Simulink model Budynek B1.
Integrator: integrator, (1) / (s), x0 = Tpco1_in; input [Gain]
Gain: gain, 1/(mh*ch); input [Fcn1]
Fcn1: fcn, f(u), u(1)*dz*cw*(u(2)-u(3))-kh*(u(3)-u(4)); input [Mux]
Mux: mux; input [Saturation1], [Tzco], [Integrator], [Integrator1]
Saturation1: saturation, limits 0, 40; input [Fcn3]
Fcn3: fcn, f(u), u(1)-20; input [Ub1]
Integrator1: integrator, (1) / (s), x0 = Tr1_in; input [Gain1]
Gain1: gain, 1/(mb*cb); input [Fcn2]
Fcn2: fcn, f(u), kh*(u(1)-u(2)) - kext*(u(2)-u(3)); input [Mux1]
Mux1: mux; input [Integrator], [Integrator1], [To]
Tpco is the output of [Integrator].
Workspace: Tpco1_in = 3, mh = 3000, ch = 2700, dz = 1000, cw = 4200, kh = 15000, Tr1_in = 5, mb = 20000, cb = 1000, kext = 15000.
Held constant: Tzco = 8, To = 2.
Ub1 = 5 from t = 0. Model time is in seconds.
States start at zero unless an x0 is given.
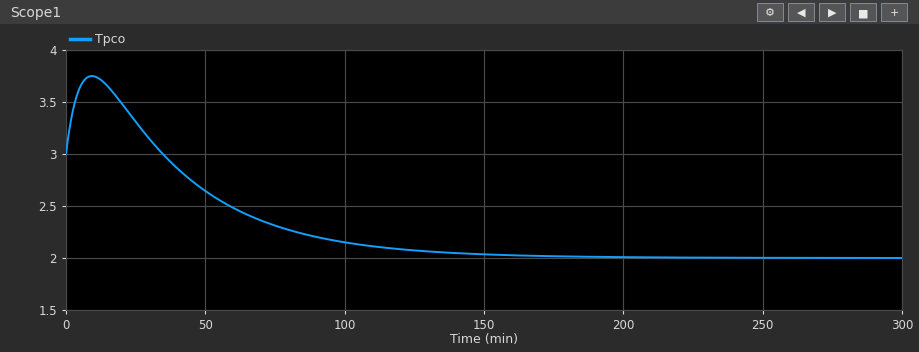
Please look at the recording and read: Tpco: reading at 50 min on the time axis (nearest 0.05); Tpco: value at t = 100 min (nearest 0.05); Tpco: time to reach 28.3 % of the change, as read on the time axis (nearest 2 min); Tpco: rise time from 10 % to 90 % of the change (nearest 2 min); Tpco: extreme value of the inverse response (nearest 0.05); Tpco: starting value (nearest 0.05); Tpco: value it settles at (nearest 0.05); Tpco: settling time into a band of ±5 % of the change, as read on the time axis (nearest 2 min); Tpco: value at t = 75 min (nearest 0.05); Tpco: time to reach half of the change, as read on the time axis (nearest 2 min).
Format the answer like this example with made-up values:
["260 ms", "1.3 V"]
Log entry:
["2.65", "2.15", "46 min", "76 min", "3.75", "3.00", "2.00", "138 min", "2.30", "58 min"]
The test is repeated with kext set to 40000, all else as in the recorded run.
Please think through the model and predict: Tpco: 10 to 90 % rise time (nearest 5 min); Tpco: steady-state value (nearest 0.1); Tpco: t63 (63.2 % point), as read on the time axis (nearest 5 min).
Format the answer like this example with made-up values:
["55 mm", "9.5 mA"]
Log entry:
["35 min", "2.0", "35 min"]
